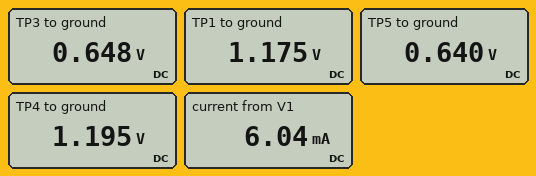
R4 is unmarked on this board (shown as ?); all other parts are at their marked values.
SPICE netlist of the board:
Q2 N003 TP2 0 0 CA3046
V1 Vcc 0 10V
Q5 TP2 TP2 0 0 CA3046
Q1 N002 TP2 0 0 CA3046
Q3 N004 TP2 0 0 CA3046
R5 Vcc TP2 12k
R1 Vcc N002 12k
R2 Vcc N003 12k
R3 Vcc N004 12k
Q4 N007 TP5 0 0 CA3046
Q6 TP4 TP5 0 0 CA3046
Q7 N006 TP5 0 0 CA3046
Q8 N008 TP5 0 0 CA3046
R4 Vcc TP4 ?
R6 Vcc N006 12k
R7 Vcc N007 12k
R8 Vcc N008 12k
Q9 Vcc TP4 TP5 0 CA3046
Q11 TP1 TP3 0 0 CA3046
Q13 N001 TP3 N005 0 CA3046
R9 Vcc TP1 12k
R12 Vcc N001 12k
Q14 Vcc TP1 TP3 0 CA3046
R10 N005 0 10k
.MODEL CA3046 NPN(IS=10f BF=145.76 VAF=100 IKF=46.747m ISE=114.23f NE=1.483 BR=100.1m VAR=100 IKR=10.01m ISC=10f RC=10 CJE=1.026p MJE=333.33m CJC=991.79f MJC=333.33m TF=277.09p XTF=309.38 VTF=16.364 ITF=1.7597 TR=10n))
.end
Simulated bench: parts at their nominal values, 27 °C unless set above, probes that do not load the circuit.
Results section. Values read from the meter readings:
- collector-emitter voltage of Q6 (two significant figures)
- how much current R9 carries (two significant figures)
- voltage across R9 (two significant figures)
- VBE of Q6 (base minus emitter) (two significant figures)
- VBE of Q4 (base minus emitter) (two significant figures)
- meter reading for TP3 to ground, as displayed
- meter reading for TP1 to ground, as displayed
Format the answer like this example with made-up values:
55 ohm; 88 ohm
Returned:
1.2 V; 740 µA; 8.8 V; 640 mV; 640 mV; 0.648 V; 1.175 V
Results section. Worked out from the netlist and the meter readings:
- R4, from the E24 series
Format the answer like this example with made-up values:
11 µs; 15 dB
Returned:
16 kΩ
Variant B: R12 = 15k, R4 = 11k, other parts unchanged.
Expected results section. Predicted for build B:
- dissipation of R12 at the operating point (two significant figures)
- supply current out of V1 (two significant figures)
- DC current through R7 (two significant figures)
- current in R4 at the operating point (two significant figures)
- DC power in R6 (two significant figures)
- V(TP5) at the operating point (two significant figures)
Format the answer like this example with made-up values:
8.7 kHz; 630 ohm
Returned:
1.8 µW; 7.0 mA; 790 µA; 800 µA; 7.5 mW; 650 mV
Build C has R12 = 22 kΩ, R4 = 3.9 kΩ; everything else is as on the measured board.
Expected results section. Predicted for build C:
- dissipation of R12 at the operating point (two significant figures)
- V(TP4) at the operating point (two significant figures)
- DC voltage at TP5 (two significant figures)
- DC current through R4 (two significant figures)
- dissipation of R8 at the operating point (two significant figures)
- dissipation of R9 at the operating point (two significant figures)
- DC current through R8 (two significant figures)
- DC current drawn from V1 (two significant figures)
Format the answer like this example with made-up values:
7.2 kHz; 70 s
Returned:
2.6 µW; 1.4 V; 680 mV; 2.2 mA; 8.2 mW; 6.5 mW; 830 µA; 12 mA
